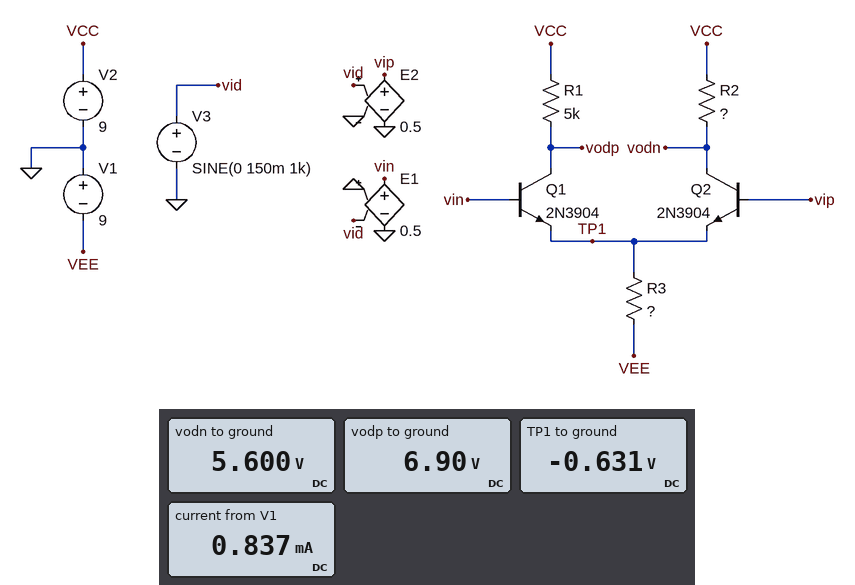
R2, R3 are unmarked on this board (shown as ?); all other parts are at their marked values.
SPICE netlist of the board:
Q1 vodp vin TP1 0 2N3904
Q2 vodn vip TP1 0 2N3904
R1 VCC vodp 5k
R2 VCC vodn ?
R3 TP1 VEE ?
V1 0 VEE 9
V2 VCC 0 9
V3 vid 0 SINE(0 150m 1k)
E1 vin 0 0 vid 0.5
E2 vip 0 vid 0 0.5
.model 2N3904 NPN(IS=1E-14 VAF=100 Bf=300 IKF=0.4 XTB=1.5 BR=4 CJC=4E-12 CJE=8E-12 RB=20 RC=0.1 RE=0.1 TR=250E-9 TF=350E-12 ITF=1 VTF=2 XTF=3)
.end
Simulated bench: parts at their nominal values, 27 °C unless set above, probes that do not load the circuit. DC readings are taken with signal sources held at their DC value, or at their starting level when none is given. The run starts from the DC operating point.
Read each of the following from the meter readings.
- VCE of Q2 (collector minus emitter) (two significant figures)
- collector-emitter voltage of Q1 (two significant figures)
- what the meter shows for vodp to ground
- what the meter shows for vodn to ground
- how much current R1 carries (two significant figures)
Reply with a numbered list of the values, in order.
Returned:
1. 6.2 V
2. 7.5 V
3. 6.90 V
4. 5.600 V
5. 420 µA
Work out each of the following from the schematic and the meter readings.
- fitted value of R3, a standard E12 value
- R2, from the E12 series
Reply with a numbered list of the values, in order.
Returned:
1. 10 kΩ
2. 8.2 kΩ
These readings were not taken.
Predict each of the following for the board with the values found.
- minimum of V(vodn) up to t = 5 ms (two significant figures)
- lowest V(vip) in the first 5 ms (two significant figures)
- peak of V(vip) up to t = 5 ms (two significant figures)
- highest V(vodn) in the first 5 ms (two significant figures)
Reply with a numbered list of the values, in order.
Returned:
1. 2.1 V
2. -75 mV
3. 75 mV
4. 9.0 V
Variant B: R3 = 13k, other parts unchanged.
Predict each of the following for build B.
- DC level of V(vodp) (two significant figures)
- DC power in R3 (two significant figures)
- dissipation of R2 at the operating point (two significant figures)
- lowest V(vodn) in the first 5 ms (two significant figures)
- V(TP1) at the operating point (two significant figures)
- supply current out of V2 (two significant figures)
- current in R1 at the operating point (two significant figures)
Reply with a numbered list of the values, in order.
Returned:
1. 7.4 V
2. 5.4 mW
3. 840 µW
4. 3.7 V
5. -620 mV
6. 640 µA
7. 320 µA
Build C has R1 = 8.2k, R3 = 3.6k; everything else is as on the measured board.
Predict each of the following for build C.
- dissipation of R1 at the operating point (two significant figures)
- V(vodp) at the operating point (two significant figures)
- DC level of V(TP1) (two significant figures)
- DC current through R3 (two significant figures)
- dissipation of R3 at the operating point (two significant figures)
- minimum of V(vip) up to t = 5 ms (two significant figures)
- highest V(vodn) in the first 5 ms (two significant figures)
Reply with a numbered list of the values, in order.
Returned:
1. 11 mW
2. -470 mV
3. -660 mV
4. 2.3 mA
5. 19 mW
6. -75 mV
7. 8.6 V
